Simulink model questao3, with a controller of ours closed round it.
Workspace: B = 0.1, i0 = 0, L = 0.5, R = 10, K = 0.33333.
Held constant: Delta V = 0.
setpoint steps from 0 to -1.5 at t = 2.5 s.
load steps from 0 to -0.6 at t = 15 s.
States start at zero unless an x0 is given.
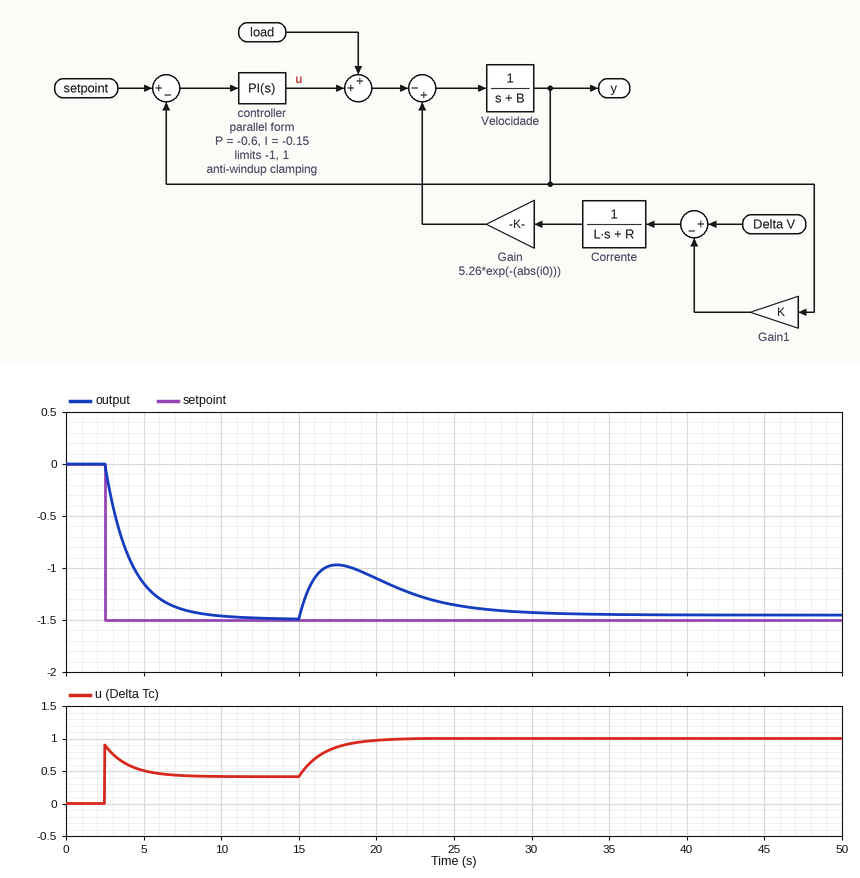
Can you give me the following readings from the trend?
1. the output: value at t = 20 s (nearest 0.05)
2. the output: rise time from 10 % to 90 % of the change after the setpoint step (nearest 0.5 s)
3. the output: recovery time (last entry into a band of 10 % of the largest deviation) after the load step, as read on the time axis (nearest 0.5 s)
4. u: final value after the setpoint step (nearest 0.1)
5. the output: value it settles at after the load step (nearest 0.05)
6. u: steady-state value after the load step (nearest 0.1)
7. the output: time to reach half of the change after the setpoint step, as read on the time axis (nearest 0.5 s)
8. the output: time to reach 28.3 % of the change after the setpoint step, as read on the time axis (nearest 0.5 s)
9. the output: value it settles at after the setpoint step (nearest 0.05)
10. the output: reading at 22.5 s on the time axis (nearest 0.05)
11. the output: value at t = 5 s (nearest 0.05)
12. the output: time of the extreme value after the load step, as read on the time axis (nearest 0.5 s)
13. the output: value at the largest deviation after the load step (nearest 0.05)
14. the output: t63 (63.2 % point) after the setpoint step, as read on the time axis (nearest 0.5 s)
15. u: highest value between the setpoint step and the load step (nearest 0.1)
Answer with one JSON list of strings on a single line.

["-1.10", "4.0 s", "27.5 s", "0.4", "-1.45", "1.0", "3.5 s", "3.0 s", "-1.50", "-1.25", "-1.15", "17.5 s", "-0.95", "4.0 s", "0.9"]
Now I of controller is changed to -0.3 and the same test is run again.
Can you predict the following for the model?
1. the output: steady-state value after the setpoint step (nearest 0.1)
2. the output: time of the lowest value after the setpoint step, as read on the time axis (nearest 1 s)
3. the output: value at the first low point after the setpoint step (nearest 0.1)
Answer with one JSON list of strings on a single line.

["-1.5", "8 s", "-1.6"]
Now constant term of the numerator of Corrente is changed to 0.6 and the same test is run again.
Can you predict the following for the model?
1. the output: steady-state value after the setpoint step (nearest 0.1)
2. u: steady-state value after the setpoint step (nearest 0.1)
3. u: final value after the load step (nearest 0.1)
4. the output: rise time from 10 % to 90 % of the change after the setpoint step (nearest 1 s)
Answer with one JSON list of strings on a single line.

["-1.5", "0.3", "0.9", "3 s"]
